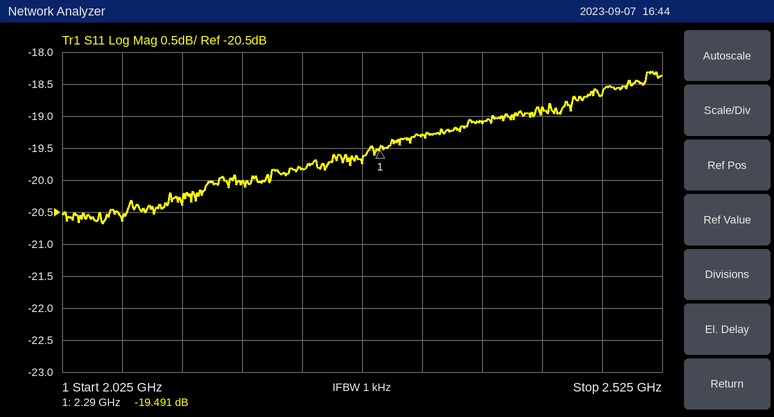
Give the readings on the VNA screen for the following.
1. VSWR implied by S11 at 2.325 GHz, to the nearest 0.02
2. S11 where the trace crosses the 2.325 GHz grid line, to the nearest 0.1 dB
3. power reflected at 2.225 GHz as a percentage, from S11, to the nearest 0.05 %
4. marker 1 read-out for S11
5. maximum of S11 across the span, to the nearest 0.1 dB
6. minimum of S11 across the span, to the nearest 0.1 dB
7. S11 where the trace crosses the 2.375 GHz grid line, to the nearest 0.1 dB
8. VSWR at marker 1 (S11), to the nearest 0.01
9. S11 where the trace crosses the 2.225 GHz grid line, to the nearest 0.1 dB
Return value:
1.24
-19.3 dB
1.05 %
-19.491 dB
-18.3 dB
-20.7 dB
-19.1 dB
1.24
-19.8 dB
